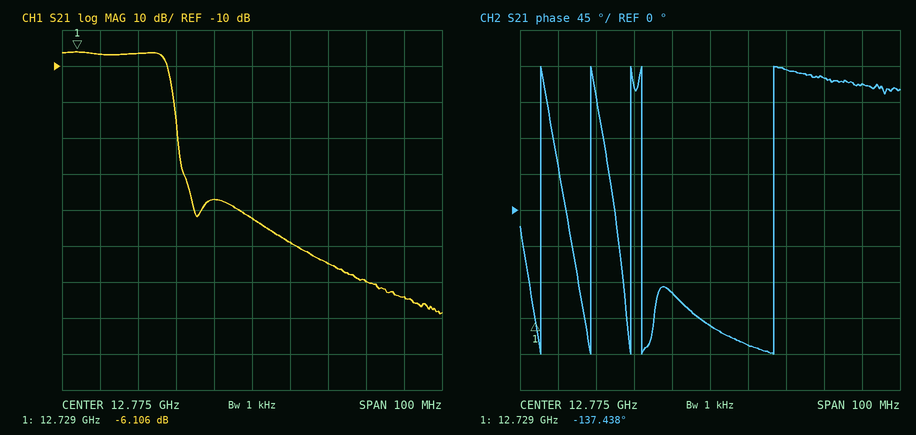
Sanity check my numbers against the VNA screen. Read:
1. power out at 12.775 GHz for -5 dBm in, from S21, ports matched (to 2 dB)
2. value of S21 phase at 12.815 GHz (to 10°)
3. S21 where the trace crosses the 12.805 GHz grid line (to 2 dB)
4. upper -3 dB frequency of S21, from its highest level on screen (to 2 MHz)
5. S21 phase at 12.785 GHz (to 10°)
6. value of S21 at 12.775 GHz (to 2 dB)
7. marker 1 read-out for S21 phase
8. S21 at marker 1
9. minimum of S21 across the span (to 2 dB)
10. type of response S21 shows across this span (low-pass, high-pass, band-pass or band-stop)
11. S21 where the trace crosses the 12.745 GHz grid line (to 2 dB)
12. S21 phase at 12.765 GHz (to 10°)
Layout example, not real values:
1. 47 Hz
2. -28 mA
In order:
1. -58 dBm
2. 160°
3. -70 dB
4. 12.752 GHz
5. -170°
6. -52 dB
7. -137.438°
8. -6.106 dB
9. -78 dB
10. low-pass
11. -6 dB
12. -100°
